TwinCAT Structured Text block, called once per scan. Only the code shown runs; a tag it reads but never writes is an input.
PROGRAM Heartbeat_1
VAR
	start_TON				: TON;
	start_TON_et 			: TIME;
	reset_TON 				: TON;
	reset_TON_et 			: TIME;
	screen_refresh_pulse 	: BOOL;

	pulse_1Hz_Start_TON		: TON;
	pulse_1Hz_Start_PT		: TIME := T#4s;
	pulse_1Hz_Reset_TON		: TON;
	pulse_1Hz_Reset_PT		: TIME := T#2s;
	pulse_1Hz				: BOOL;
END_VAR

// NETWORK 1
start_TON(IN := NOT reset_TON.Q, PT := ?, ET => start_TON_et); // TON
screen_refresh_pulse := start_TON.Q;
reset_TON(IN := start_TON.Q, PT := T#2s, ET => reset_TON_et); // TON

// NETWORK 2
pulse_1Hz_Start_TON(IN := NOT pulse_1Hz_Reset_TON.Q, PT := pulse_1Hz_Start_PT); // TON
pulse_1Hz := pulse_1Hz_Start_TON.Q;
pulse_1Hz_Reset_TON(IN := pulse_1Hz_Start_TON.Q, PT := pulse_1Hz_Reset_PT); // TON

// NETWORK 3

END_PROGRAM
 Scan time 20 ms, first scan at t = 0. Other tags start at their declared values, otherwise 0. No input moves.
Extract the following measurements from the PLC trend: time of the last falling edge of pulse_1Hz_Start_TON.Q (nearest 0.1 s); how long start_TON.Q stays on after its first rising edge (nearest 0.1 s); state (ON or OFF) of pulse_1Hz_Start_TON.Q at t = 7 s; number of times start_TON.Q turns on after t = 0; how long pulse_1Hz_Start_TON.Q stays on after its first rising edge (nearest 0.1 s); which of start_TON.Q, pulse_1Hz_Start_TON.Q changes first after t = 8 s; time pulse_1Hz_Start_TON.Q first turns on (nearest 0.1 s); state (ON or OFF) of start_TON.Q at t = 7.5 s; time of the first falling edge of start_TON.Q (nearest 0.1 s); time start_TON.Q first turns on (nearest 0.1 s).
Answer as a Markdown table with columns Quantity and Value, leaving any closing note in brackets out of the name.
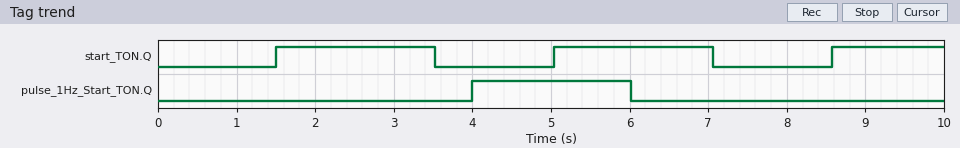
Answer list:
| Quantity | Value |
|---|---|
| time of the last falling edge of pulse_1Hz_Start_TON.Q | 6.0 s |
| how long start_TON.Q stays on after its first rising edge | 2.0 s |
| state (ON or OFF) of pulse_1Hz_Start_TON.Q at t = 7 s | OFF |
| number of times start_TON.Q turns on after t = 0 | 3 |
| how long pulse_1Hz_Start_TON.Q stays on after its first rising edge | 2.0 s |
| which of start_TON.Q, pulse_1Hz_Start_TON.Q changes first after t = 8 s | start_TON.Q |
| time pulse_1Hz_Start_TON.Q first turns on | 4.0 s |
| state (ON or OFF) of start_TON.Q at t = 7.5 s | OFF |
| time of the first falling edge of start_TON.Q | 3.5 s |
| time start_TON.Q first turns on | 1.5 s |
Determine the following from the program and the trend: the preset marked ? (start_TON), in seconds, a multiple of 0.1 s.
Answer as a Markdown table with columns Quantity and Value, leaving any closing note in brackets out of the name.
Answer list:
| Quantity | Value |
|---|---|
| the preset marked ? (start_TON), in seconds, a multiple of 0.1 s | 1.5 s |
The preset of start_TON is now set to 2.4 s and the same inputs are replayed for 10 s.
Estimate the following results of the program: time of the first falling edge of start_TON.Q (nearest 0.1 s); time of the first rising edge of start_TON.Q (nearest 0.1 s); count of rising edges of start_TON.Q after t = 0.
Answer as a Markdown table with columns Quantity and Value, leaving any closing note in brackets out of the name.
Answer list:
| Quantity | Value |
|---|---|
| time of the first falling edge of start_TON.Q | 4.4 s |
| time of the first rising edge of start_TON.Q | 2.4 s |
| count of rising edges of start_TON.Q after t = 0 | 2 |
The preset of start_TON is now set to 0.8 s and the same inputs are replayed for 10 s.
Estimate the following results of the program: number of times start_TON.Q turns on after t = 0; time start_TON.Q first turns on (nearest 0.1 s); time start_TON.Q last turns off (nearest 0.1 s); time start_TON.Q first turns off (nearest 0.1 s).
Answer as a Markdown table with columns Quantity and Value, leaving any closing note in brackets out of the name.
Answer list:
| Quantity | Value |
|---|---|
| number of times start_TON.Q turns on after t = 0 | 4 |
| time start_TON.Q first turns on | 0.8 s |
| time start_TON.Q last turns off | 8.5 s |
| time start_TON.Q first turns off | 2.8 s |
